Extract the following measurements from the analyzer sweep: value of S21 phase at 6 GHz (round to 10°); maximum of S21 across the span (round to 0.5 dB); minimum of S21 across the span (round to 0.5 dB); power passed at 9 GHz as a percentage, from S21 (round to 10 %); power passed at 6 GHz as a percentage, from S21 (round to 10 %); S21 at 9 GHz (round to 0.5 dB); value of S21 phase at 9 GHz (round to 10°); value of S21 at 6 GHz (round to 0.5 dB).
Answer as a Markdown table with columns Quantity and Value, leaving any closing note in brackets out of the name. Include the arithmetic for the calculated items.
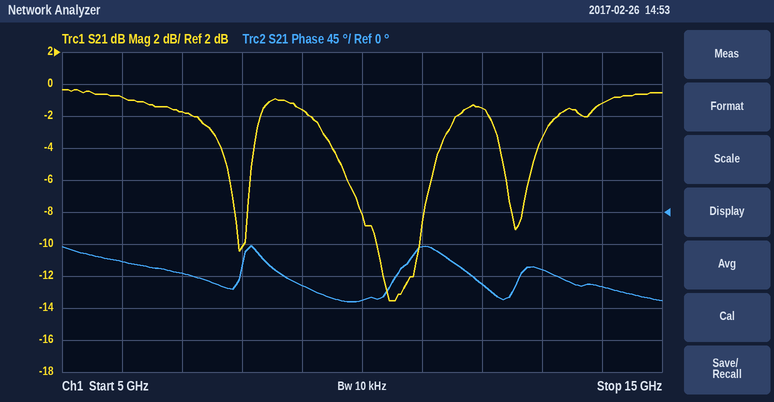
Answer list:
| Quantity | Value |
|---|---|
| value of S21 phase at 6 GHz | -70° |
| maximum of S21 across the span | -0.5 dB |
| minimum of S21 across the span | -13.5 dB |
| power passed at 9 GHz as a percentage, from S21 | 10^(-1.5/10) ≈ 70.8 %, so 70 % to the nearest 10 % |
| power passed at 6 GHz as a percentage, from S21 | 10^(-1/10) ≈ 79.4 %, so 80 % to the nearest 10 % |
| S21 at 9 GHz | -1.5 dB |
| value of S21 phase at 9 GHz | -100° |
| value of S21 at 6 GHz | -1.0 dB |
